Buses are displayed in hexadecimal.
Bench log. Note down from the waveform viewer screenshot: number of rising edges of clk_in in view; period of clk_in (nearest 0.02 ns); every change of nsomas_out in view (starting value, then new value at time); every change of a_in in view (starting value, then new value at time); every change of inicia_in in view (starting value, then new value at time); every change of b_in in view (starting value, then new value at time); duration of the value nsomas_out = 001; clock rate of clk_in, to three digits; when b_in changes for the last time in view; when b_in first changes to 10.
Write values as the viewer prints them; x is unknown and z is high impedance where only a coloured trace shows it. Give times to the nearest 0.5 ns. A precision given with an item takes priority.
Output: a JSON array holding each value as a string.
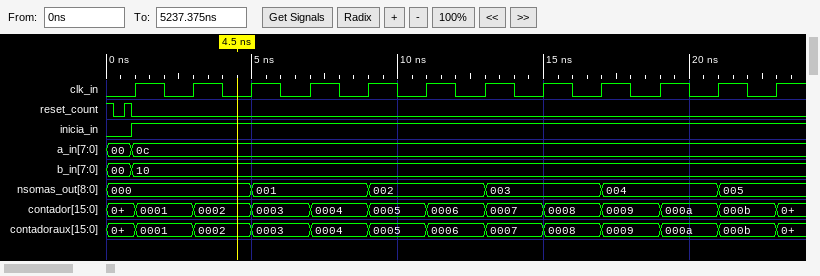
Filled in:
["12", "2 ns", "000, 001 at 5 ns, 002 at 9 ns, 003 at 13 ns, 004 at 17 ns, 005 at 21 ns", "00, 0c at 1 ns", "0, 1 at 1 ns", "00, 10 at 1 ns", "4 ns", "500 MHz", "1 ns", "1 ns"]
